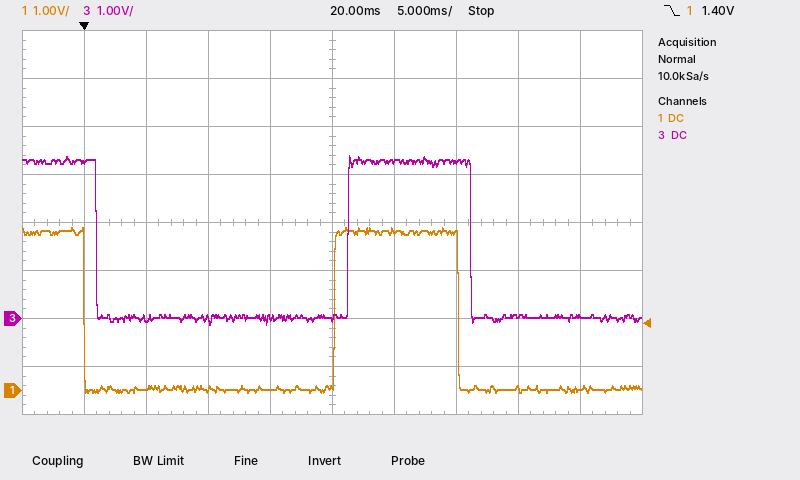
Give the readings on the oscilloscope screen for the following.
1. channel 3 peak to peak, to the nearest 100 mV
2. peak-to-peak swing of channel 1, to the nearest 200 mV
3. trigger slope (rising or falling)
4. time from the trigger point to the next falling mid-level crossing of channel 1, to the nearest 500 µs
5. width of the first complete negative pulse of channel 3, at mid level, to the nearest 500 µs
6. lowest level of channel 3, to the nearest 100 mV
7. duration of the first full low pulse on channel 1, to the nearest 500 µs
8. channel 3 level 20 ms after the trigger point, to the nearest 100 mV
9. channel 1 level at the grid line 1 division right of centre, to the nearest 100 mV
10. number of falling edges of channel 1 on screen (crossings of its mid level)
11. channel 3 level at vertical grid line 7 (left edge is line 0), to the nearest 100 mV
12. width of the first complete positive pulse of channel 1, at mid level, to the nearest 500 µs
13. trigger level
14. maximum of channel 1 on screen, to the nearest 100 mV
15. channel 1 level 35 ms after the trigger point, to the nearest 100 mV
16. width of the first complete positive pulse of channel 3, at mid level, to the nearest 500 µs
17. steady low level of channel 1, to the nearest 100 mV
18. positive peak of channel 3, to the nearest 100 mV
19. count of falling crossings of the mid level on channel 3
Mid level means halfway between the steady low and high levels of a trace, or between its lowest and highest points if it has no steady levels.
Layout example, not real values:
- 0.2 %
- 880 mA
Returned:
- 3.5 V
- 3.4 V
- falling
- 30.0 ms
- 20.5 ms
- -100 mV
- 20.0 ms
- 0.0 V
- 3.3 V
- 2
- 3.3 V
- 10.0 ms
- 1.40 V
- 3.4 V
- 0.0 V
- 10.0 ms
- 0.0 V
- 3.4 V
- 2
